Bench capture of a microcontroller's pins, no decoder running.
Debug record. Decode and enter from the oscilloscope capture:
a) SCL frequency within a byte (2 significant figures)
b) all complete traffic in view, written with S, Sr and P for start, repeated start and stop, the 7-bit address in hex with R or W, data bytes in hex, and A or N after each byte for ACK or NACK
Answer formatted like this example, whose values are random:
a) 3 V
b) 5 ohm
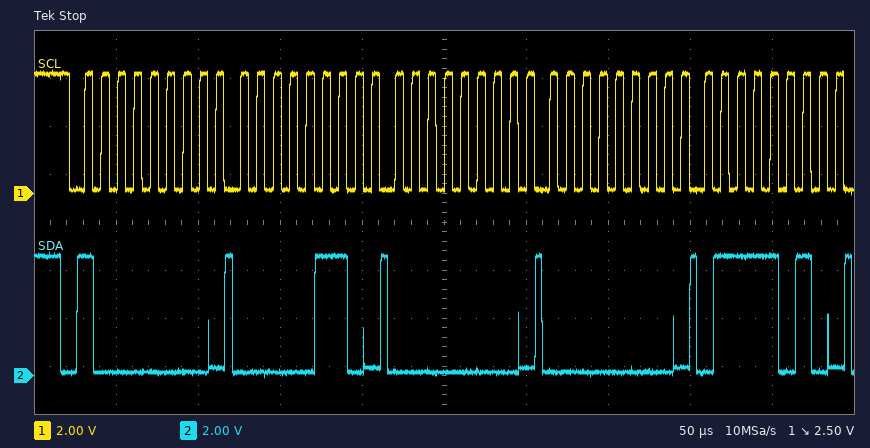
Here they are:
a) 100 kHz
b) S 40W A 06 A 00 A 00 A 7A A
